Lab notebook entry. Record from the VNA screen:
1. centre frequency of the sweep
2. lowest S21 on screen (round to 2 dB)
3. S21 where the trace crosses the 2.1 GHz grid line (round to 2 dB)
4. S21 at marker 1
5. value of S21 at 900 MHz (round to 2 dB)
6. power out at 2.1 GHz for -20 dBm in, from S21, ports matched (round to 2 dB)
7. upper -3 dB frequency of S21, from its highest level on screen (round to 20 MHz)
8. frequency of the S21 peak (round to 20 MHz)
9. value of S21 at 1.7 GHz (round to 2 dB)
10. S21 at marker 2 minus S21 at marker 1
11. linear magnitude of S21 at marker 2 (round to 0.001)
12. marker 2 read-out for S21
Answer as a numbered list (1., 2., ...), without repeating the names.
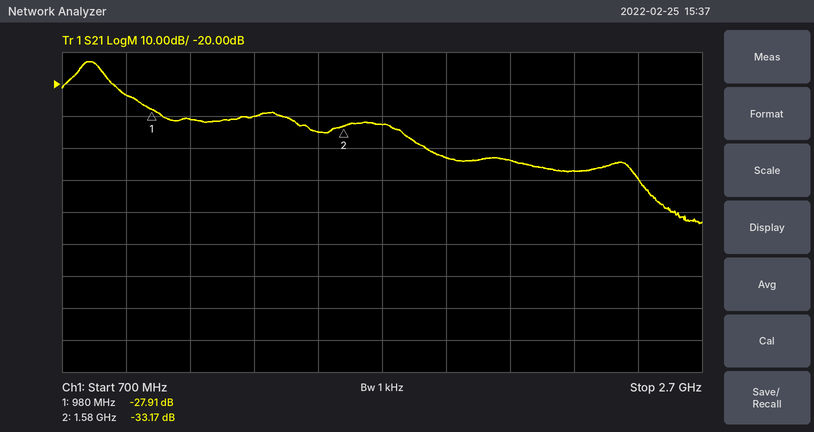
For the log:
1. 1.7 GHz
2. -64 dB
3. -44 dB
4. -27.91 dB
5. -24 dB
6. -64 dBm
7. 820 MHz
8. 780 MHz
9. -32 dB
10. -5.26 dB
11. 0.022
12. -33.17 dB
